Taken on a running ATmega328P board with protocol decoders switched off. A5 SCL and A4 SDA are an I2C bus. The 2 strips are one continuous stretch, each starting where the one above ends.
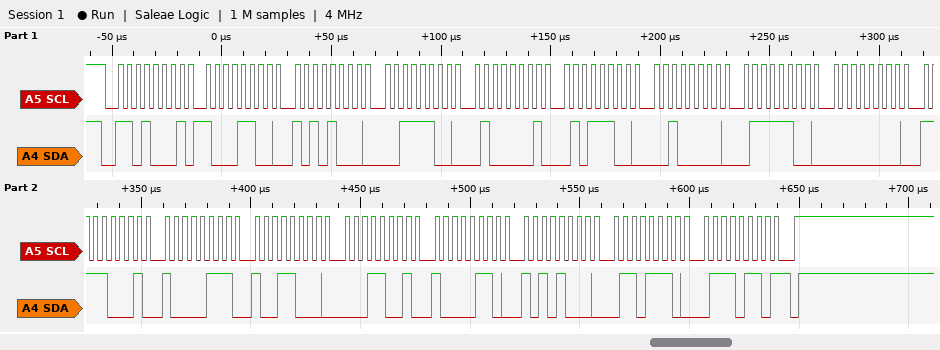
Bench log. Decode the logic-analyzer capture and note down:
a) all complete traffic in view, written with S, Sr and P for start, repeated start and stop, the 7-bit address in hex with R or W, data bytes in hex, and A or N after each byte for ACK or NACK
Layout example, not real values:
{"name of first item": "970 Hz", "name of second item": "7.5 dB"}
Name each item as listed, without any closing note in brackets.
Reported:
{"all complete traffic in view, written with S, Sr and P for start, repeated start and stop, the 7-bit address in hex with R or W, data bytes in hex, and A or N after each byte for ACK or NACK": "S 68R A 8C A A8 A 3C A 41 A 5C A 20 A 7C A 00 A F1 A 87 A 98 A 19 A 86 A A8 A 6E A 76 N P"}
